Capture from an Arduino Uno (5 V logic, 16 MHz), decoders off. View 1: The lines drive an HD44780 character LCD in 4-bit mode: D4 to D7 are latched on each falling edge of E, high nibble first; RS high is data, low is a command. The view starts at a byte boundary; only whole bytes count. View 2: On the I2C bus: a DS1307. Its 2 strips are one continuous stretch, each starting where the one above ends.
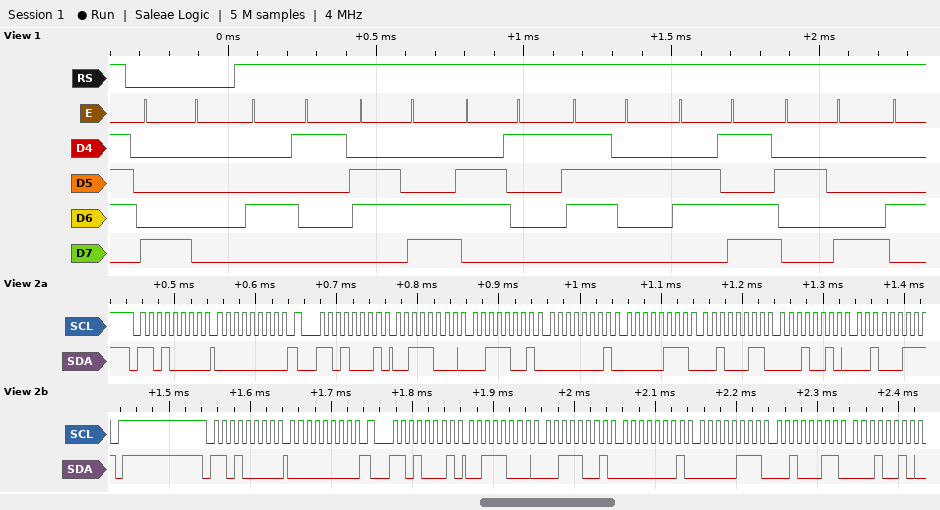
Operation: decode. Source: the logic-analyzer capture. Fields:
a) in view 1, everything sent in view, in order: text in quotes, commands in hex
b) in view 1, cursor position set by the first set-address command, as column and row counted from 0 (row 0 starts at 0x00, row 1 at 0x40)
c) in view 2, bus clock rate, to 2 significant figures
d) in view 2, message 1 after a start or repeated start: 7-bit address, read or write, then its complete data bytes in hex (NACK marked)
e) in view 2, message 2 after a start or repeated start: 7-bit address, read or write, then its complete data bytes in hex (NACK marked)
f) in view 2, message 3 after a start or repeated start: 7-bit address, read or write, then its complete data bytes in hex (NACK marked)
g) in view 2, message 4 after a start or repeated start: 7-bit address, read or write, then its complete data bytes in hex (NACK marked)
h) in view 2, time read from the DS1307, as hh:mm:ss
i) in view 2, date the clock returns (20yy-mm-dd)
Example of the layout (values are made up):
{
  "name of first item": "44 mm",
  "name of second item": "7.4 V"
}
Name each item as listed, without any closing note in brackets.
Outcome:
{
  "in view 1, everything sent in view, in order: text in quotes, commands in hex": "0x80 \"Alarm(\"",
  "in view 1, cursor position set by the first set-address command, as column and row counted from 0": "column 0, row 0",
  "in view 2, bus clock rate, to 2 significant figures": "100 kHz",
  "in view 2, message 1 after a start or repeated start: 7-bit address, read or write, then its complete data bytes in hex": "0x68 write: 00",
  "in view 2, message 2 after a start or repeated start: 7-bit address, read or write, then its complete data bytes in hex": "0x68 read: 38 39 01 07 23 12 23 NACK",
  "in view 2, message 3 after a start or repeated start: 7-bit address, read or write, then its complete data bytes in hex": "0x68 write: 00",
  "in view 2, message 4 after a start or repeated start: 7-bit address, read or write, then its complete data bytes in hex": "0x68 read: 38 39 01 07 23 12",
  "in view 2, time read from the DS1307, as hh:mm:ss": "01:39:38",
  "in view 2, date the clock returns": "2023-12-23"
}
